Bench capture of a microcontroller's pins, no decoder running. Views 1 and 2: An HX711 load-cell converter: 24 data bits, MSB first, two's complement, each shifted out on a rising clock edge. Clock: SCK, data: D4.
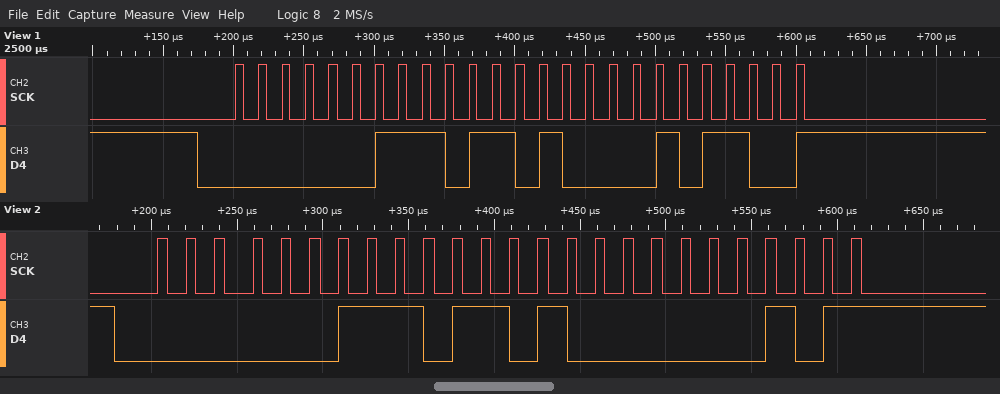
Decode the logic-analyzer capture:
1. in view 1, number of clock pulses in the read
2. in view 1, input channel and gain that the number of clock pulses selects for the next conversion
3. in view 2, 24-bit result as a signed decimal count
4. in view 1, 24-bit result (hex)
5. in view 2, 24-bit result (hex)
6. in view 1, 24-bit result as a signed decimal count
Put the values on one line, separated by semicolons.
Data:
25; channel A, gain 128; 242693; 0x03B42C; 0x03B405; 242732
